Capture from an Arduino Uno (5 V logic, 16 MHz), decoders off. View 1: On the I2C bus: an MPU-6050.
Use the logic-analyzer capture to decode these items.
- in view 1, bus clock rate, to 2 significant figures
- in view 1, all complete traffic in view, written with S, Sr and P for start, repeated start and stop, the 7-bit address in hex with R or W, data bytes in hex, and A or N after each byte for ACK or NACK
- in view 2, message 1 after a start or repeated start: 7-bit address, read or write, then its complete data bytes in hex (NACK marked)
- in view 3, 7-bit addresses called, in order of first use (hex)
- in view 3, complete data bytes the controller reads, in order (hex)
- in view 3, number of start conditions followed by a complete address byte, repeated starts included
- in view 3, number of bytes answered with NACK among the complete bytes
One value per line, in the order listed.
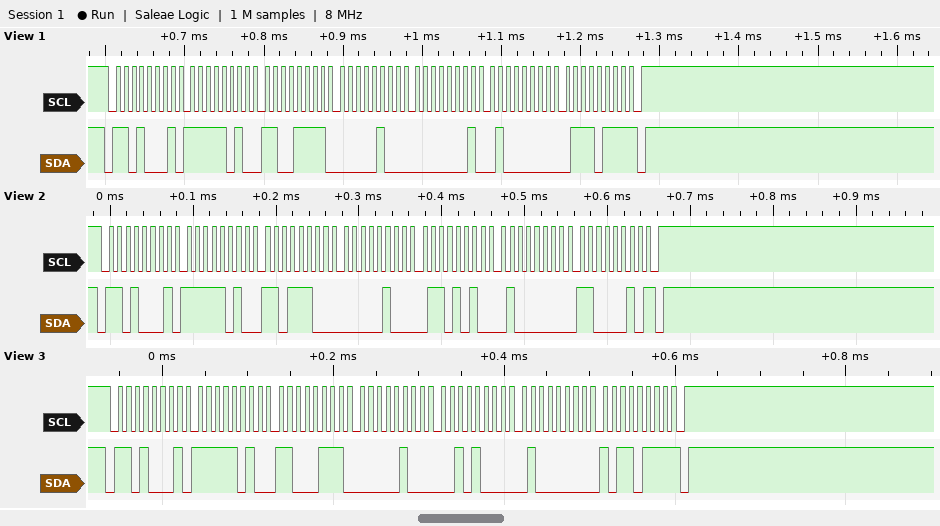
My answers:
100 kHz
S 68R A FA A CF A 04 A 01 A 40 A 77 N P
0x68 read: FA DC 04 6A 40 C2 NACK
0x68
FA C7 04 28 40 B7
1
1
